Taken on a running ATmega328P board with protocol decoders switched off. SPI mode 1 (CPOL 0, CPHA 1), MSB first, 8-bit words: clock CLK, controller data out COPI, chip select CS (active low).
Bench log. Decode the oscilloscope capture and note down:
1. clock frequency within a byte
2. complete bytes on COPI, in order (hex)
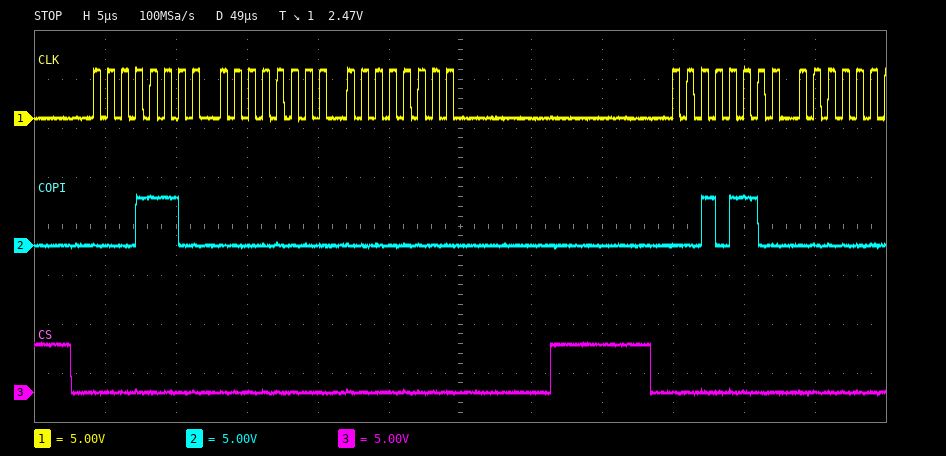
1 MHz
1C 00 00 2C
